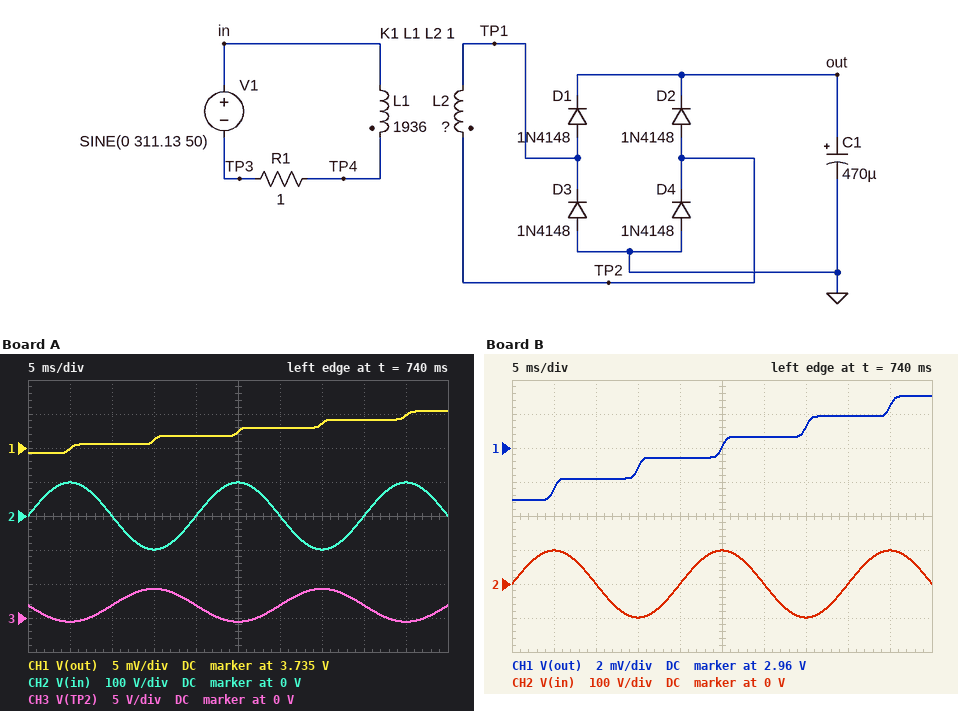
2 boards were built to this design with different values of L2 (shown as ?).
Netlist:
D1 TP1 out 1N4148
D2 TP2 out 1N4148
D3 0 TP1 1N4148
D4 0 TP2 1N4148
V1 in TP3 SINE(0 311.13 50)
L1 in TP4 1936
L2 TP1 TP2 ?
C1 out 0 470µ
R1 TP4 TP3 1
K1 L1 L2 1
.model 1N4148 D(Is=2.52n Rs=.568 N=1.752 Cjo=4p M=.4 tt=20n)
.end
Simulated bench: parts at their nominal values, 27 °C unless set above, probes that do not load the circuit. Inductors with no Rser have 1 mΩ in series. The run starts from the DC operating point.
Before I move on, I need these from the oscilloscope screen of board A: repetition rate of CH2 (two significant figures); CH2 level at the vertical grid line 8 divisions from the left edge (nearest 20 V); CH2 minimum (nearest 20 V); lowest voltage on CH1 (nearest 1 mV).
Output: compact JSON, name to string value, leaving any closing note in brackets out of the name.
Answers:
{"repetition rate of CH2": "50 Hz", "CH2 level at the vertical grid line 8 divisions from the left edge": "0 V", "CH2 minimum": "-100 V", "lowest voltage on CH1": "3.734 V"}
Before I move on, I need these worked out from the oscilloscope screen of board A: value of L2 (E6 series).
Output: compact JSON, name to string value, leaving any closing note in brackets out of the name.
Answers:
{"value of L2": "470 mH"}
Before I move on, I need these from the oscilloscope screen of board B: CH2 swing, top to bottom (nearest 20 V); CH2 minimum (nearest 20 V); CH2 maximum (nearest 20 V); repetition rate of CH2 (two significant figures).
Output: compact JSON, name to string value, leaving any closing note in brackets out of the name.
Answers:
{"CH2 swing, top to bottom": "200 V", "CH2 minimum": "-100 V", "CH2 maximum": "100 V", "repetition rate of CH2": "50 Hz"}
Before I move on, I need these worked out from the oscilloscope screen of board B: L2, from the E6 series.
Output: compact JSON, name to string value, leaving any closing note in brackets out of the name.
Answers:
{"L2, from the E6 series": "330 mH"}
